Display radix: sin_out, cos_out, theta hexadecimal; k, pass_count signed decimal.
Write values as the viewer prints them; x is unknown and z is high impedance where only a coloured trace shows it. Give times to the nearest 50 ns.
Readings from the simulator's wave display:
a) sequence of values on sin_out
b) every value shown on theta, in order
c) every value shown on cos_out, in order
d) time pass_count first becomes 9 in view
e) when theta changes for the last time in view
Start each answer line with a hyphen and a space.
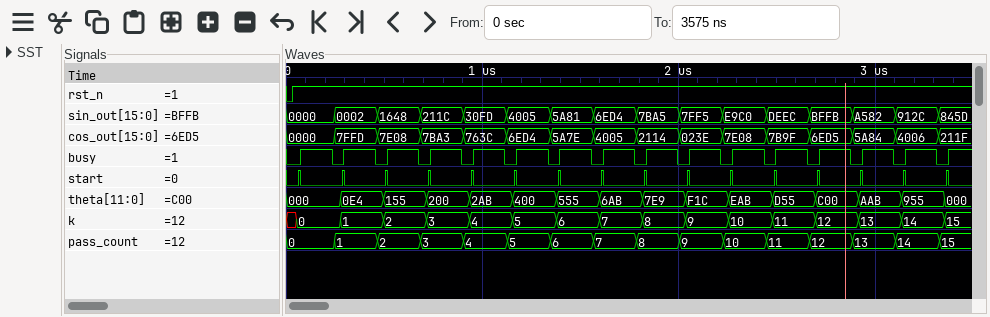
- 0000, 0002, 1648, 211C, 30FD, 4005, 5A81, 6ED4, 7BA5, 7FF5, E9C0, DEEC, BFFB, A582, 912C, 845D
- 000, 0E4, 155, 200, 2AB, 400, 555, 6AB, 7E9, F1C, EAB, D55, C00, AAB, 955, 000
- 0000, 7FFD, 7E08, 7BA3, 763C, 6ED4, 5A7E, 4005, 2114, 023E, 7E08, 7B9F, 6ED5, 5A84, 4006, 211F
- 2000 ns
- 3350 ns
